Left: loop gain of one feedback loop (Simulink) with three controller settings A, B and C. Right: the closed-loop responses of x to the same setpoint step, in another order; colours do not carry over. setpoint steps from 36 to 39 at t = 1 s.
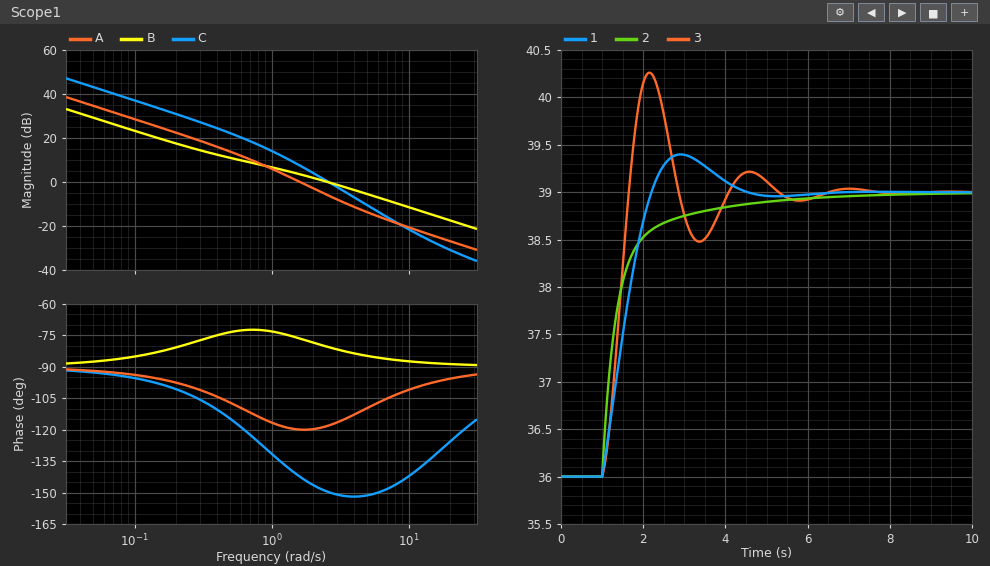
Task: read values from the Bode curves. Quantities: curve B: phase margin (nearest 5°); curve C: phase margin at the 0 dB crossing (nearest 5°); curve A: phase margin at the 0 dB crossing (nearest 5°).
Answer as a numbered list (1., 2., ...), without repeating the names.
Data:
1. 100°
2. 30°
3. 60°
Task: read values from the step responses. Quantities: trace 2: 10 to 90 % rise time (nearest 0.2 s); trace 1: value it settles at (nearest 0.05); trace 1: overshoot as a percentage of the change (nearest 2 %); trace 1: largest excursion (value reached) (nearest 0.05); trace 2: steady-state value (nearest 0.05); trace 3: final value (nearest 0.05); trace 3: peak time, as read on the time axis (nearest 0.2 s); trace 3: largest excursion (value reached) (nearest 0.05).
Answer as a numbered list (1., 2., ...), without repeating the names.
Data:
1. 1.6 s
2. 39.00
3. 14 %
4. 39.40
5. 39.00
6. 39.00
7. 2.2 s
8. 40.25
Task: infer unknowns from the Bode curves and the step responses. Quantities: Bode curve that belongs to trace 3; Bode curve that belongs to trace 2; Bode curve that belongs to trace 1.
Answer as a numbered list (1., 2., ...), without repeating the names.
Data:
1. C
2. B
3. A
